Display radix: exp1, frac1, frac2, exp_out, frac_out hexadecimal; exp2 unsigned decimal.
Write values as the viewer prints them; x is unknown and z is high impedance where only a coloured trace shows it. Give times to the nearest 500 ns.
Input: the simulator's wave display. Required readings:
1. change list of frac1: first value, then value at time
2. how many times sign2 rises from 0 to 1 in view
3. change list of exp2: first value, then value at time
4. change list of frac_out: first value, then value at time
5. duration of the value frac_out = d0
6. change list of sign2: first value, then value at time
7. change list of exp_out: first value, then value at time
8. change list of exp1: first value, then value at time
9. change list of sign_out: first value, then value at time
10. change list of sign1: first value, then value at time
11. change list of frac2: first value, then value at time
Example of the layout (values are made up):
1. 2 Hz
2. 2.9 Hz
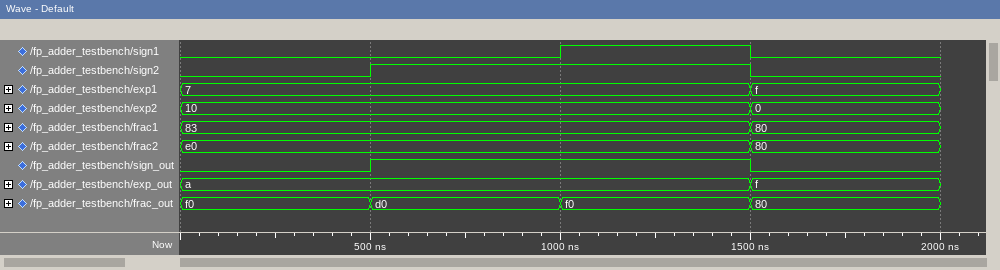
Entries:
1. 83, 80 at 1500 ns
2. 1
3. 10, 0 at 1500 ns
4. f0, d0 at 500 ns, f0 at 1000 ns, 80 at 1500 ns
5. 500 ns
6. 0, 1 at 500 ns, 0 at 1500 ns
7. a, f at 1500 ns
8. 7, f at 1500 ns
9. 0, 1 at 500 ns, 0 at 1500 ns
10. 0, 1 at 1000 ns, 0 at 1500 ns
11. e0, 80 at 1500 ns
